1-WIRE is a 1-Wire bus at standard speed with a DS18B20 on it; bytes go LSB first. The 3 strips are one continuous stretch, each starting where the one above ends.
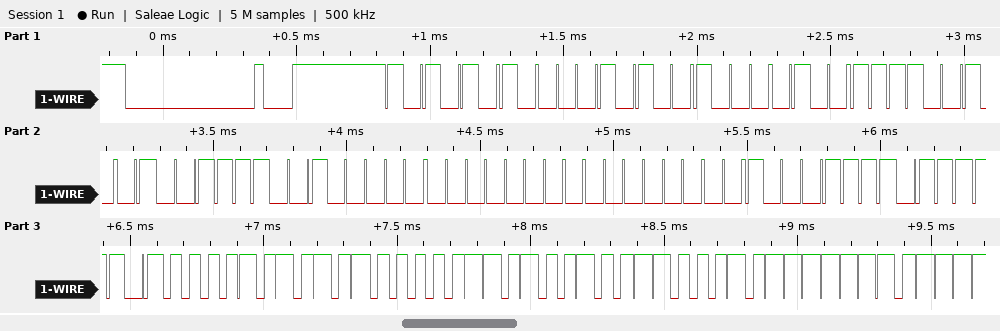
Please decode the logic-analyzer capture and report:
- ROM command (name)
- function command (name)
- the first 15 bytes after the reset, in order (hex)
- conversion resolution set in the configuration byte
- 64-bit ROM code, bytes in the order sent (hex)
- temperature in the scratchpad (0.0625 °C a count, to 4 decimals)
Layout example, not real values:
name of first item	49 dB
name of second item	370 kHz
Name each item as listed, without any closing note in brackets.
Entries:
ROM command	Match ROM
function command	Read Scratchpad
the first 15 bytes after the reset, in order	55 28 21 4F F2 04 00 00 F1 BE 50 05 4B 46 7F
conversion resolution set in the configuration byte	12 bits
64-bit ROM code, bytes in the order sent	28 21 4F F2 04 00 00 F1
temperature in the scratchpad	85.0000 °C
